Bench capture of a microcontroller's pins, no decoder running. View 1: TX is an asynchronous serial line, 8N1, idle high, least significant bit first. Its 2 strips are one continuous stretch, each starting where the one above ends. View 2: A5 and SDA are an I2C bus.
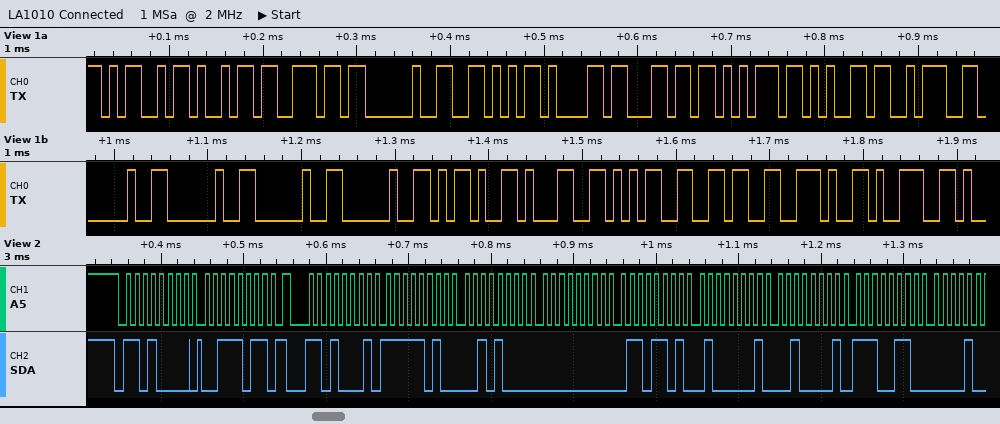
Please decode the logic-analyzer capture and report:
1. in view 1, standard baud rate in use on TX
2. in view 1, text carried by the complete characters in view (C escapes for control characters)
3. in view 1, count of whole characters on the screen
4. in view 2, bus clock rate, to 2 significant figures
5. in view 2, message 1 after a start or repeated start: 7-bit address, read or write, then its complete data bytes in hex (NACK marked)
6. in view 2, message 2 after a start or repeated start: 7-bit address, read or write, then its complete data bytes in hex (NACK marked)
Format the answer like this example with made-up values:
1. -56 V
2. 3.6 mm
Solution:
1. 115200 baud
2. "Min Value:    -156.9"
3. 20
4. 100 kHz
5. 0x68 write: 3B
6. 0x68 read: FA 28 00 6D 41 21 E6
